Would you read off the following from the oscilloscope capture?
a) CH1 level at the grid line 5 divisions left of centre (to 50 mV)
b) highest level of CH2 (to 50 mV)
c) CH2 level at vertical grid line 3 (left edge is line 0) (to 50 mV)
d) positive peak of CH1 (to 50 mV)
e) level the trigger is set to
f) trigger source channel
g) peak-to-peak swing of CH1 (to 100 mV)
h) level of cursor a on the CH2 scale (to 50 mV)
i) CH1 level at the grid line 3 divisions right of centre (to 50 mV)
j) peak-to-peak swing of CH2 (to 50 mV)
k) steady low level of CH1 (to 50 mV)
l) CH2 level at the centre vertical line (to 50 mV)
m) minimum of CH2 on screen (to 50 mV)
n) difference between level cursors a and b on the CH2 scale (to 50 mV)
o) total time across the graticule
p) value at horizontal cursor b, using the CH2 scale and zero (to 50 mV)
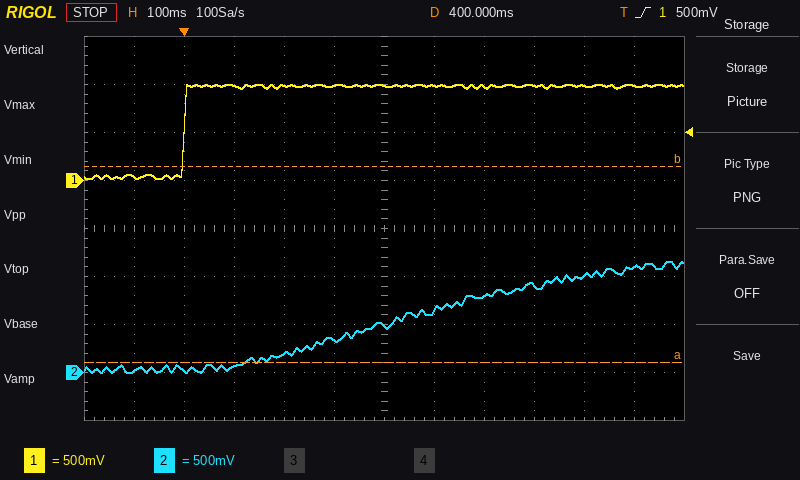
50 mV
1.15 V
50 mV
1.00 V
500 mV
CH1
1.00 V
100 mV
1.00 V
1.15 V
50 mV
500 mV
0 mV
2.05 V
1.2 s
2.15 V
